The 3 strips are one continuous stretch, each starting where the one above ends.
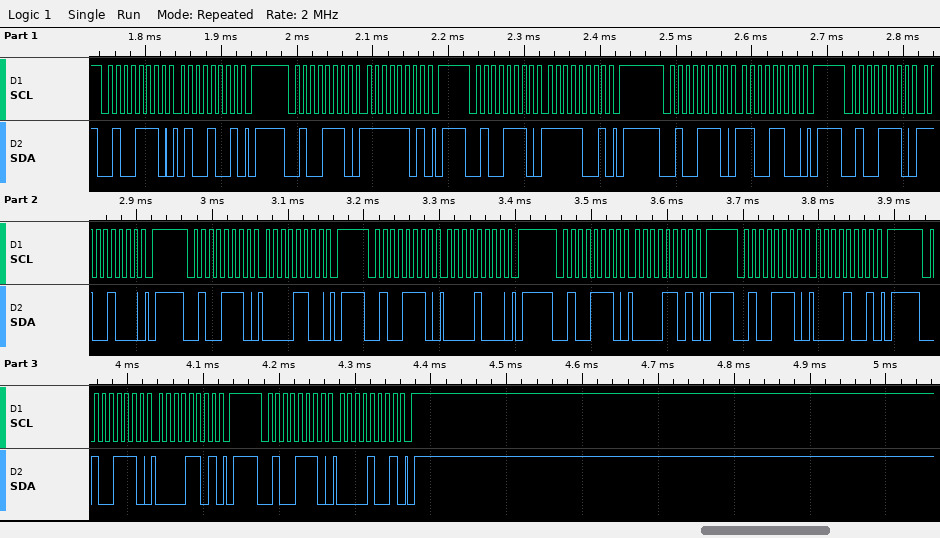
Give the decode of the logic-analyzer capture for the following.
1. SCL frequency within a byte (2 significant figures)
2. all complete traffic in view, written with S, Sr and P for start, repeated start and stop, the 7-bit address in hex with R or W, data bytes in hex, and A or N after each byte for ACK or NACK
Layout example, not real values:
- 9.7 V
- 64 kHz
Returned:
- 100 kHz
- S 27W A 49 A P S 27W A FD A P S 27W A F9 A P S 27W A CC A P S 27W A C8 A P S 27W A 0C A P S 27W A 08 A P S 27W A 0D A P S 27W A 09 A P S 27W A 0D A P S 27W A 09 A P
